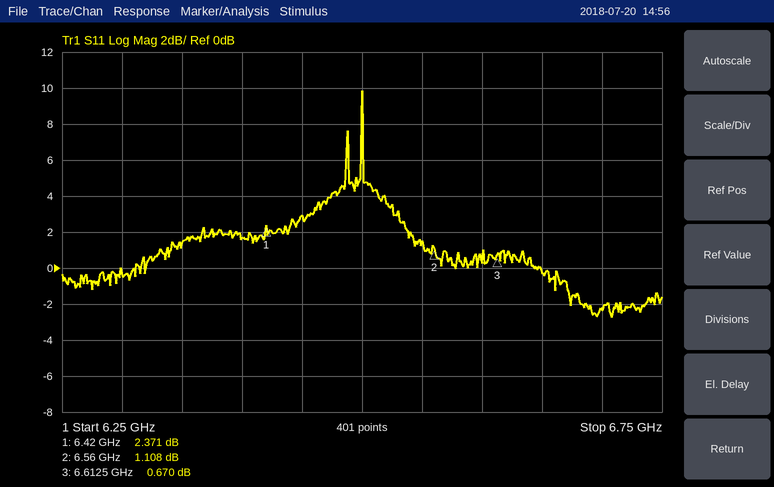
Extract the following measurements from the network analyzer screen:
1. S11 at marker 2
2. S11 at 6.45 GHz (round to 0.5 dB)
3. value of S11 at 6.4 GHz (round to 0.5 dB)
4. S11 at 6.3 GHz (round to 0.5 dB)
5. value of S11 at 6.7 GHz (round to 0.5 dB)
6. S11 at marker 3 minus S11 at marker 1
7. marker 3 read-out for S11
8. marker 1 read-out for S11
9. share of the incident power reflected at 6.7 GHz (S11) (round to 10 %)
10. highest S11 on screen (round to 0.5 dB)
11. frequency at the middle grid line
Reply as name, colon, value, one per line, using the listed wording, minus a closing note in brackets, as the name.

S11 at marker 2: 1.108 dB
S11 at 6.45 GHz: 3.0 dB
value of S11 at 6.4 GHz: 1.5 dB
S11 at 6.3 GHz: -0.5 dB
value of S11 at 6.7 GHz: -2.5 dB
S11 at marker 3 minus S11 at marker 1: -1.701 dB
marker 3 read-out for S11: 0.670 dB
marker 1 read-out for S11: 2.371 dB
share of the incident power reflected at 6.7 GHz (S11): 60 %
highest S11 on screen: 10.0 dB
frequency at the middle grid line: 6.5 GHz
